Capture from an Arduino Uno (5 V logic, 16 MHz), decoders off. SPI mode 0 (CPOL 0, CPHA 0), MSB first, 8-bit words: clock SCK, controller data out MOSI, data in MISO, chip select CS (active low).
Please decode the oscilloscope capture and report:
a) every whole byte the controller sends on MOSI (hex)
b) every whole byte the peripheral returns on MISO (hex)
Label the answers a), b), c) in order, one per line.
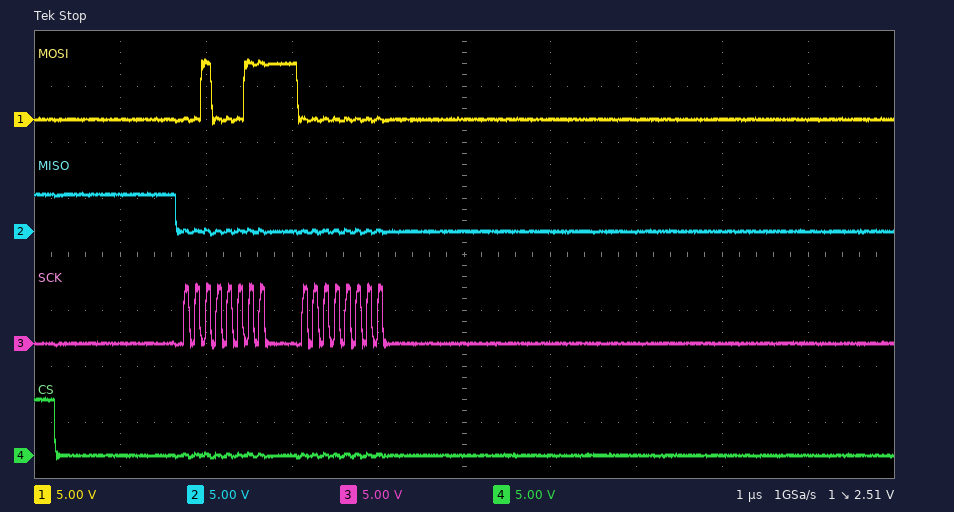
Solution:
a) 0x23 0x00
b) 0x00 0x00
